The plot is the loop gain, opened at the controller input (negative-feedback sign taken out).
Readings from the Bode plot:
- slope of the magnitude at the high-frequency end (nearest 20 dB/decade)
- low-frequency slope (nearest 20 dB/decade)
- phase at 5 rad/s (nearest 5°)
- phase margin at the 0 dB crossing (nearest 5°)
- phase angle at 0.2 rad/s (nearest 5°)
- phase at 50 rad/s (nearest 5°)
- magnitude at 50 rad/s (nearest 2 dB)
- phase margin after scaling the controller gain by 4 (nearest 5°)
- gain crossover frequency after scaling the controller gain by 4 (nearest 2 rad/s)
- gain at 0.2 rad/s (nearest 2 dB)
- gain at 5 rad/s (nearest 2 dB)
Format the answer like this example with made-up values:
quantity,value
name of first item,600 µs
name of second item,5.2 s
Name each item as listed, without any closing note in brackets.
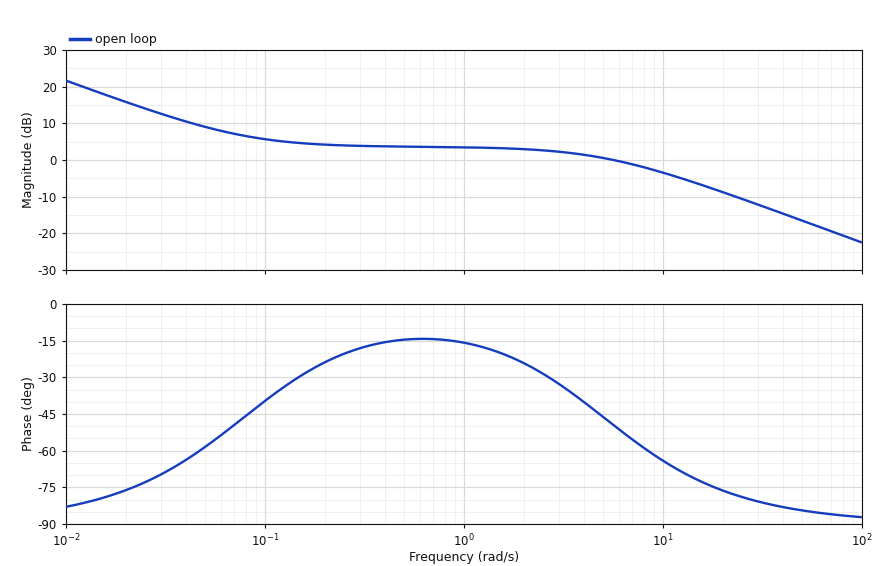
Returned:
quantity,value
slope of the magnitude at the high-frequency end,-20 dB/decade
low-frequency slope,-20 dB/decade
phase at 5 rad/s,-45°
phase margin at the 0 dB crossing,130°
phase angle at 0.2 rad/s,-25°
phase at 50 rad/s,-85°
magnitude at 50 rad/s,-16 dB
phase margin after scaling the controller gain by 4,100°
gain crossover frequency after scaling the controller gain by 4,30 rad/s
gain at 0.2 rad/s,4 dB
gain at 5 rad/s,0 dB
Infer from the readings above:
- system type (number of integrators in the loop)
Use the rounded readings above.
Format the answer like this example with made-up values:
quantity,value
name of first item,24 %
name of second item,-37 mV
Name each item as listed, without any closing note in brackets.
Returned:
quantity,value
system type,1
